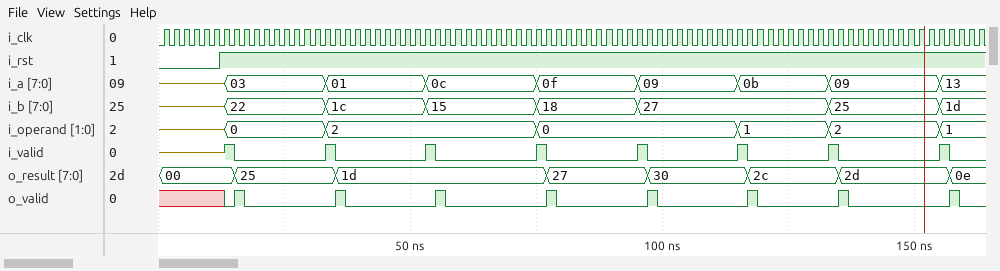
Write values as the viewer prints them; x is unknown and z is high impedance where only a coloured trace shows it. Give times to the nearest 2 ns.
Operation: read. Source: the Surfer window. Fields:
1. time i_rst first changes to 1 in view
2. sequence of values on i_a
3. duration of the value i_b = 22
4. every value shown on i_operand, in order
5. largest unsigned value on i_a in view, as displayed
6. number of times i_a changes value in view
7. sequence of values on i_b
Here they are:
12 ns
z, 03, 01, 0c, 0f, 09, 0b, 09, 13
20 ns
z, 0, 2, 0, 1, 2, 1
13
8
z, 22, 1c, 15, 18, 27, 25, 1d
